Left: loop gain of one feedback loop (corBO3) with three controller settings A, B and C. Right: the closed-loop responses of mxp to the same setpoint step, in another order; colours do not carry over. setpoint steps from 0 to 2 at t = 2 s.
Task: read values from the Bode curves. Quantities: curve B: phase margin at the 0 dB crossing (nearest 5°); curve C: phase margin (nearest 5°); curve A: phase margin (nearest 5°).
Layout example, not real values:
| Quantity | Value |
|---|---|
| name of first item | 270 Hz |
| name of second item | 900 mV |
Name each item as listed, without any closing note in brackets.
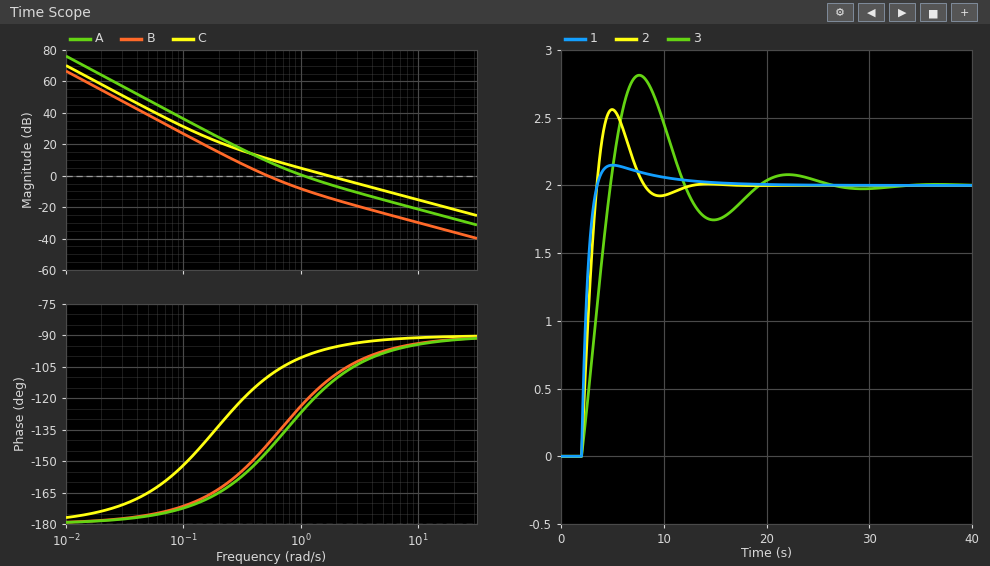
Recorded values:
| Quantity | Value |
|---|---|
| curve B: phase margin at the 0 dB crossing | 40° |
| curve C: phase margin | 85° |
| curve A: phase margin | 55° |
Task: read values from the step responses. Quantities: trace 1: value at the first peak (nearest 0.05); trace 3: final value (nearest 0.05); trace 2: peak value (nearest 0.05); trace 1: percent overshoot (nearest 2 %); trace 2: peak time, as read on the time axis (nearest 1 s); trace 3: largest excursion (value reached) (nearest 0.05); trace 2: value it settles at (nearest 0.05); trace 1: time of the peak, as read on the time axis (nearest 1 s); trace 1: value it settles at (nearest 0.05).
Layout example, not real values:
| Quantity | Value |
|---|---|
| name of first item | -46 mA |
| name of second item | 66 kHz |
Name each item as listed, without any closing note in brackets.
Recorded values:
| Quantity | Value |
|---|---|
| trace 1: value at the first peak | 2.15 |
| trace 3: final value | 2.00 |
| trace 2: peak value | 2.55 |
| trace 1: percent overshoot | 8 % |
| trace 2: peak time, as read on the time axis | 5 s |
| trace 3: largest excursion (value reached) | 2.80 |
| trace 2: value it settles at | 2.00 |
| trace 1: time of the peak, as read on the time axis | 5 s |
| trace 1: value it settles at | 2.00 |
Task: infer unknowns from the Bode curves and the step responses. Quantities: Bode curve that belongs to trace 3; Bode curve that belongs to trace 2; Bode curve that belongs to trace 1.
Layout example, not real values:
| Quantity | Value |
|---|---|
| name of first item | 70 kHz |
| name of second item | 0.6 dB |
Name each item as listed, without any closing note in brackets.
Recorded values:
| Quantity | Value |
|---|---|
| Bode curve that belongs to trace 3 | B |
| Bode curve that belongs to trace 2 | A |
| Bode curve that belongs to trace 1 | C |
